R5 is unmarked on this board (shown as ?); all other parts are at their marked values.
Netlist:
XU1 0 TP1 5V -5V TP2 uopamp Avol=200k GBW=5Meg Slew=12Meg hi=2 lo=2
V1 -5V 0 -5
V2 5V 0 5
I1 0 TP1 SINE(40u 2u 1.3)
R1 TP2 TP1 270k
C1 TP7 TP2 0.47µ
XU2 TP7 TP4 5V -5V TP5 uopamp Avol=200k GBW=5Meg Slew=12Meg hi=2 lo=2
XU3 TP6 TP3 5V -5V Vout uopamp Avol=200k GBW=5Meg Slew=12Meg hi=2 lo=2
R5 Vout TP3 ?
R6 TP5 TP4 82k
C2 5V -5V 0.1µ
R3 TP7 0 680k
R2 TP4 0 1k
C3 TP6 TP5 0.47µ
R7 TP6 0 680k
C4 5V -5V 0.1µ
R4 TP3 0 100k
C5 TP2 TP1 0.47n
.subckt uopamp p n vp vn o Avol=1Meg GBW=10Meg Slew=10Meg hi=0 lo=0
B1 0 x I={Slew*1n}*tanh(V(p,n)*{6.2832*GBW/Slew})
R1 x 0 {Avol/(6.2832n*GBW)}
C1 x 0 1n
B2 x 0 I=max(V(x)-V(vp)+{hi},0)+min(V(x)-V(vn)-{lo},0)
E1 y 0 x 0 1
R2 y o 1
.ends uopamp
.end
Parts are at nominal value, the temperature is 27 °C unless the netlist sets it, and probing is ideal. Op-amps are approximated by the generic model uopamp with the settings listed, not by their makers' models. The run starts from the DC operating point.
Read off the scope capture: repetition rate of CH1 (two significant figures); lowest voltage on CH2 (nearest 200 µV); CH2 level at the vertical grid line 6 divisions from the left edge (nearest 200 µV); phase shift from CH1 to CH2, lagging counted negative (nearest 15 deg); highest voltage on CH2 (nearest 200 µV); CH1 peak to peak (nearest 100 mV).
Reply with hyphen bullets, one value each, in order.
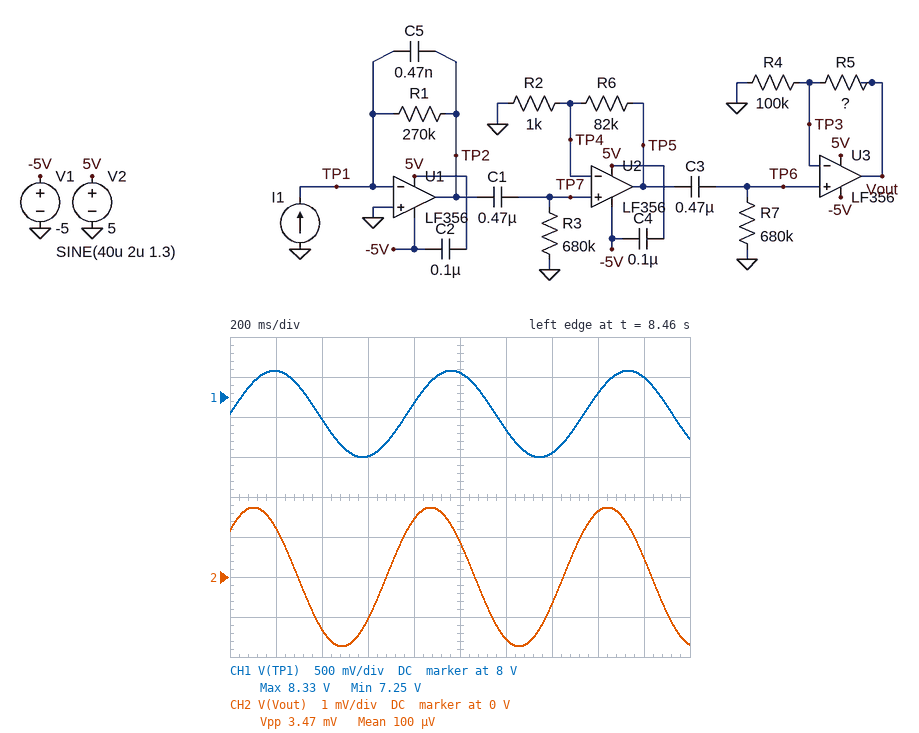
- 1.3 Hz
- -1.8 mV
- -1.6 mV
- 45 deg
- 1.8 mV
- 1.1 V
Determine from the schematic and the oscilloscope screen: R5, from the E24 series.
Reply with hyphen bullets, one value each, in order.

- 1.1 MΩ
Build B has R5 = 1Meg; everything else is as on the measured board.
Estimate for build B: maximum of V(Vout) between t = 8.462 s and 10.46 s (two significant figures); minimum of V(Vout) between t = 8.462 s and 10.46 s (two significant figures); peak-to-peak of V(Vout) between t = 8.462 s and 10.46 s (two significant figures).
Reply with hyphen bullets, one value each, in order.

- 1.6 mV
- -1.6 mV
- 3.2 mV
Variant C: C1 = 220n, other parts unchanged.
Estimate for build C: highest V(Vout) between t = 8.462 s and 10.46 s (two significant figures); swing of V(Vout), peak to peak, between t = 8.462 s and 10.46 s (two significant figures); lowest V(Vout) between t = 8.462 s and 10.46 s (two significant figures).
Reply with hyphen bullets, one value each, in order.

- 1.4 mV
- 2.9 mV
- -1.4 mV
